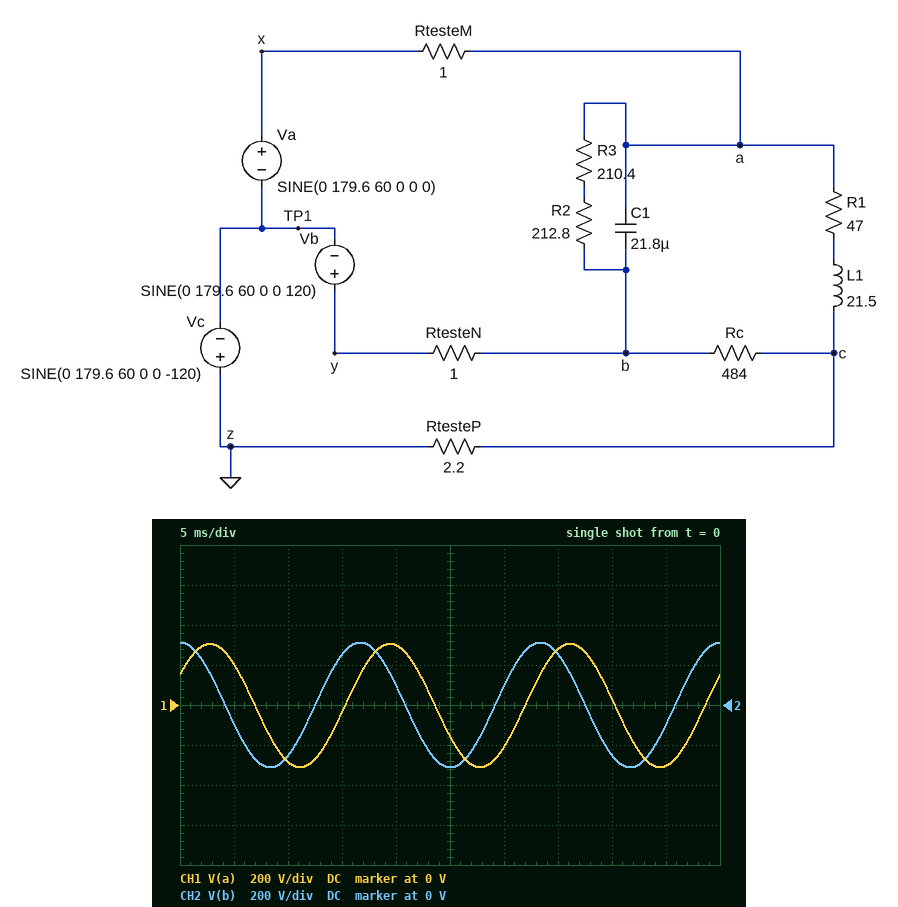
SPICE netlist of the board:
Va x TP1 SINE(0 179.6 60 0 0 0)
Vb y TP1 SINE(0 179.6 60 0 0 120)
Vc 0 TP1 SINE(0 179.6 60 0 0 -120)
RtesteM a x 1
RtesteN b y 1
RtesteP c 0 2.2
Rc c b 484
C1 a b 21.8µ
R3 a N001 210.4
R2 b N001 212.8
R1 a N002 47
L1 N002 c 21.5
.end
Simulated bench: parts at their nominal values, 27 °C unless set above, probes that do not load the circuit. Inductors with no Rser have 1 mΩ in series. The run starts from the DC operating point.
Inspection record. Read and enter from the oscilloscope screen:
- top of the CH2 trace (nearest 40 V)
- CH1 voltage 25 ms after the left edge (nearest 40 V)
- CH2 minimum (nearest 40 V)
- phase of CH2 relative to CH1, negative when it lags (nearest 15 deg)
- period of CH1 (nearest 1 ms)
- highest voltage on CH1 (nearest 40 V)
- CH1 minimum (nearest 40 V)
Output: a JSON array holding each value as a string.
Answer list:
["320 V", "-160 V", "-320 V", "60 deg", "17 ms", "320 V", "-320 V"]
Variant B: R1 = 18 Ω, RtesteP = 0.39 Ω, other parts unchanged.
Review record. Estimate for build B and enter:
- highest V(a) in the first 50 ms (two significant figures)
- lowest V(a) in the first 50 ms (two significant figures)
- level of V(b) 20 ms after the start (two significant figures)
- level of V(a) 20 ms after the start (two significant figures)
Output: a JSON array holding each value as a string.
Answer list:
["300 V", "-320 V", "98 V", "290 V"]
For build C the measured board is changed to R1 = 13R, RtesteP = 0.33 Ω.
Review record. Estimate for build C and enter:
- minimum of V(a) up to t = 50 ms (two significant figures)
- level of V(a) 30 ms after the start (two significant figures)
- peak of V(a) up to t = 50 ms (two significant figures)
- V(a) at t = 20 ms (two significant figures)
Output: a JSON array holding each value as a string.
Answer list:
["-320 V", "-220 V", "300 V", "290 V"]
